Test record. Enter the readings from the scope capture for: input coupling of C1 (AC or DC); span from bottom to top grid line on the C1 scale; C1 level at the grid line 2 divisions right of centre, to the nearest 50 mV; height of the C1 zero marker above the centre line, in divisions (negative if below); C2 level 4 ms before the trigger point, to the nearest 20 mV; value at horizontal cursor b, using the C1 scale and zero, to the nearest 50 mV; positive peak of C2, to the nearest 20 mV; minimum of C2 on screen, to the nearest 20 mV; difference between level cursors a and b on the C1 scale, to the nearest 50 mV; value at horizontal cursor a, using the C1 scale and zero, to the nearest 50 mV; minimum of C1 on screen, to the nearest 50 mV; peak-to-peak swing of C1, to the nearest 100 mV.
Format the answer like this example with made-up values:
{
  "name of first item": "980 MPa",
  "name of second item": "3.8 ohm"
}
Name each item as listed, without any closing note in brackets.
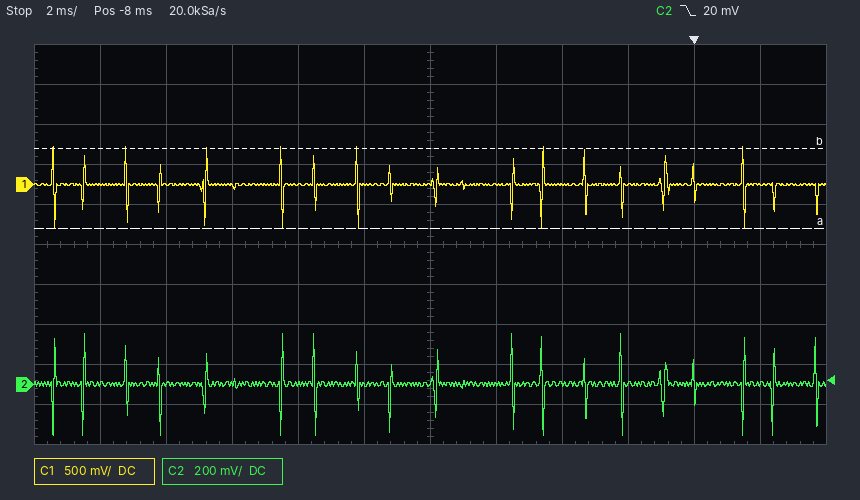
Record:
{
  "input coupling of C1": "DC",
  "span from bottom to top grid line on the C1 scale": "5 V",
  "C1 level at the grid line 2 divisions right of centre, to the nearest 50 mV": "0 mV",
  "height of the C1 zero marker above the centre line, in divisions": "+1.5 div",
  "C2 level 4 ms before the trigger point, to the nearest 20 mV": "0 mV",
  "value at horizontal cursor b, using the C1 scale and zero, to the nearest 50 mV": "450 mV",
  "positive peak of C2, to the nearest 20 mV": "260 mV",
  "minimum of C2 on screen, to the nearest 20 mV": "-260 mV",
  "difference between level cursors a and b on the C1 scale, to the nearest 50 mV": "1.00 V",
  "value at horizontal cursor a, using the C1 scale and zero, to the nearest 50 mV": "-550 mV",
  "minimum of C1 on screen, to the nearest 50 mV": "-550 mV",
  "peak-to-peak swing of C1, to the nearest 100 mV": "1.00 V"
}
